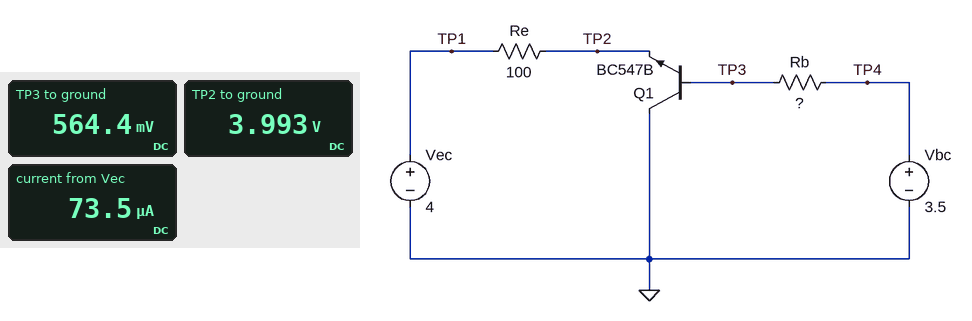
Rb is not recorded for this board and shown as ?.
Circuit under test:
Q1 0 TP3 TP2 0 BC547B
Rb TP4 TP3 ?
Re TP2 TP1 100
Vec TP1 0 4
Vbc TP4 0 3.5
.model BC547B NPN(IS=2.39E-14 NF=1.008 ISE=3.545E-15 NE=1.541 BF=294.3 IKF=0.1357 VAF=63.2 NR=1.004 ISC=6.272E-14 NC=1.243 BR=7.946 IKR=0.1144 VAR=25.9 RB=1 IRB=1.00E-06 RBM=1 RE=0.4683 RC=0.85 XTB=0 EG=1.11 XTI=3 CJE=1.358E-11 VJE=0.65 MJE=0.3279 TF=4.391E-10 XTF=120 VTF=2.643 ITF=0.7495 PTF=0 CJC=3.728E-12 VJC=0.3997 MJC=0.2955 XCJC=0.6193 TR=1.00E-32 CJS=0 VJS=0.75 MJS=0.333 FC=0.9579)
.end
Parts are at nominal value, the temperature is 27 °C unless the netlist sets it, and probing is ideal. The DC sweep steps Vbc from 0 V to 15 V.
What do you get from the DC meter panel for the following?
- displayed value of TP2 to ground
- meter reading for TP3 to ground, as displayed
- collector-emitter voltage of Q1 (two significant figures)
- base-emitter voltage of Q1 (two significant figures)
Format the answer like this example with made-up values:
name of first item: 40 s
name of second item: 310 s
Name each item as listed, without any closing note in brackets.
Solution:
displayed value of TP2 to ground: 3.993 V
meter reading for TP3 to ground, as displayed: 564.4 mV
collector-emitter voltage of Q1: -4.0 V
base-emitter voltage of Q1: -3.4 V
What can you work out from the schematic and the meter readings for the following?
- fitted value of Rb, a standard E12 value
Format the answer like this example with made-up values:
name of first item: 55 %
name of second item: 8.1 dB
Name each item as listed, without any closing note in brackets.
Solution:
fitted value of Rb, a standard E12 value: 270 kΩ
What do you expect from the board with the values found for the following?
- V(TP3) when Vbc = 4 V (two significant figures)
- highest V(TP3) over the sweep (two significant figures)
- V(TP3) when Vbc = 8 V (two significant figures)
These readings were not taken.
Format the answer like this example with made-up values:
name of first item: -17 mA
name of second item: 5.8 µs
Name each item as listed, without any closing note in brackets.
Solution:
V(TP3) when Vbc = 4 V: 570 mV
highest V(TP3) over the sweep: 610 mV
V(TP3) when Vbc = 8 V: 590 mV
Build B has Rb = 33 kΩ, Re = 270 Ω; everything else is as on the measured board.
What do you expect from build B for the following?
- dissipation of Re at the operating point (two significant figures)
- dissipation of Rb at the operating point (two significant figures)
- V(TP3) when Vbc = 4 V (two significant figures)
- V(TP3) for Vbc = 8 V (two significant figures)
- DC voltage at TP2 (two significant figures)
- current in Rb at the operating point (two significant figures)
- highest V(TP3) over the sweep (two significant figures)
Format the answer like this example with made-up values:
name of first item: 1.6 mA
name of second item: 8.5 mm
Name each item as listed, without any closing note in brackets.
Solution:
dissipation of Re at the operating point: 110 µW
dissipation of Rb at the operating point: 250 µW
V(TP3) when Vbc = 4 V: 630 mV
V(TP3) for Vbc = 8 V: 650 mV
DC voltage at TP2: 3.8 V
current in Rb at the operating point: 87 µA
highest V(TP3) over the sweep: 670 mV
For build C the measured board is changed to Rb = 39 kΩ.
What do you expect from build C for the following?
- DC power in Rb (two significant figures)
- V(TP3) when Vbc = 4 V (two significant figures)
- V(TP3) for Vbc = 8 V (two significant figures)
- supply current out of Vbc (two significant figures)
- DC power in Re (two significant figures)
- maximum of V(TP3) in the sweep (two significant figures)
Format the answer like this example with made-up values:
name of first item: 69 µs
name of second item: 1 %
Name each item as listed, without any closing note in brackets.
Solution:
DC power in Rb: 210 µW
V(TP3) when Vbc = 4 V: 620 mV
V(TP3) for Vbc = 8 V: 640 mV
supply current out of Vbc: 74 µA
DC power in Re: 29 µW
maximum of V(TP3) in the sweep: 660 mV
